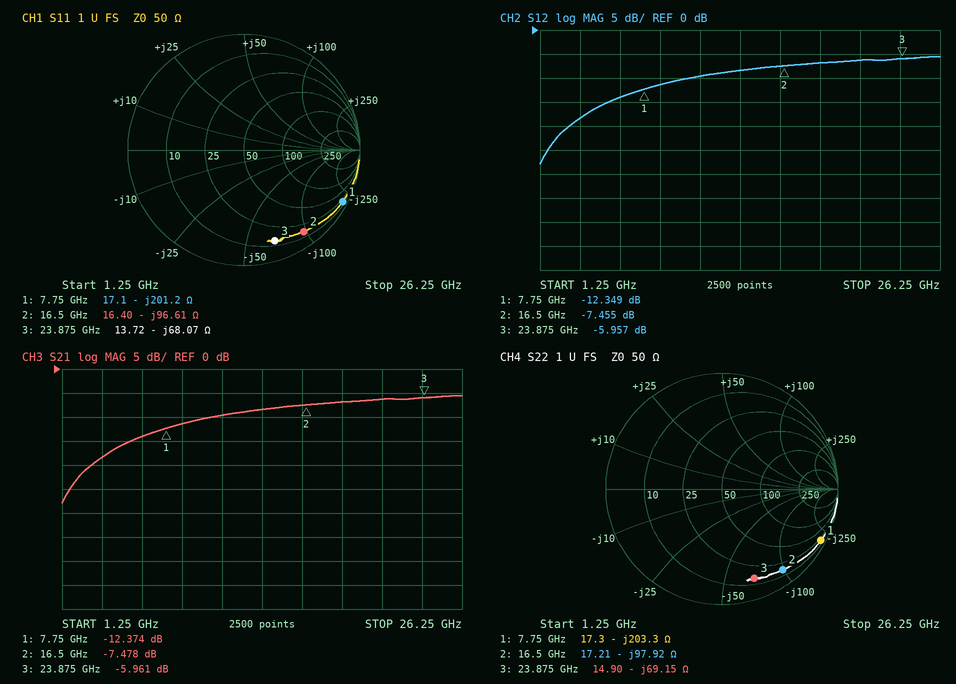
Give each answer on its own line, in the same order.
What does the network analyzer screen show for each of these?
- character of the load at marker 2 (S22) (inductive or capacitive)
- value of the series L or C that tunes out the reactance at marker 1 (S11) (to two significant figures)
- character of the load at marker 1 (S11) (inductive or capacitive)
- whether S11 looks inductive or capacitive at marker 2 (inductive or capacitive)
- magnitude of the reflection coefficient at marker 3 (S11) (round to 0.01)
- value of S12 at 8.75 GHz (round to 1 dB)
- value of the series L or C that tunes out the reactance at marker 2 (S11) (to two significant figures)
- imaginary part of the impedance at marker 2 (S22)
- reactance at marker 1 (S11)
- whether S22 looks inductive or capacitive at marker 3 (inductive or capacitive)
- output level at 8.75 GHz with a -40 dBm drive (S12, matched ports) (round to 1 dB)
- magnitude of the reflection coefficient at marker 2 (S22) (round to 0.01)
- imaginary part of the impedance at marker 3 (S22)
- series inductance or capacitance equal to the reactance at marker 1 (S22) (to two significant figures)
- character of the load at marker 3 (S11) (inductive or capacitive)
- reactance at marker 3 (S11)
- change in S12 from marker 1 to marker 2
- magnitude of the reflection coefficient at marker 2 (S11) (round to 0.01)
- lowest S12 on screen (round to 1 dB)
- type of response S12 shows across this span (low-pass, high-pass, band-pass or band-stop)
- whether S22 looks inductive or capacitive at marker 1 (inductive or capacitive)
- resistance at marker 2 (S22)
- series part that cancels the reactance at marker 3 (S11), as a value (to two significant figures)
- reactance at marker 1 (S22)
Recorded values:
capacitive
4.1 nH
capacitive
capacitive
0.83
-11 dB
930 pH
-97.92 Ω
-201.2 Ω
capacitive
-51 dBm
0.87
-69.15 Ω
100 fF
capacitive
-68.07 Ω
4.894 dB
0.87
-28 dB
high-pass
capacitive
17.21 Ω
450 pH
-203.3 Ω
